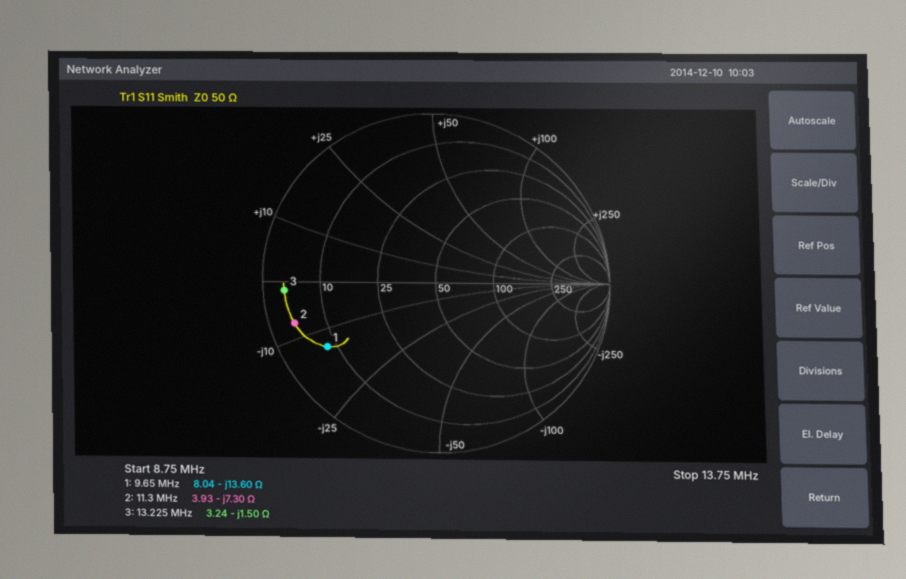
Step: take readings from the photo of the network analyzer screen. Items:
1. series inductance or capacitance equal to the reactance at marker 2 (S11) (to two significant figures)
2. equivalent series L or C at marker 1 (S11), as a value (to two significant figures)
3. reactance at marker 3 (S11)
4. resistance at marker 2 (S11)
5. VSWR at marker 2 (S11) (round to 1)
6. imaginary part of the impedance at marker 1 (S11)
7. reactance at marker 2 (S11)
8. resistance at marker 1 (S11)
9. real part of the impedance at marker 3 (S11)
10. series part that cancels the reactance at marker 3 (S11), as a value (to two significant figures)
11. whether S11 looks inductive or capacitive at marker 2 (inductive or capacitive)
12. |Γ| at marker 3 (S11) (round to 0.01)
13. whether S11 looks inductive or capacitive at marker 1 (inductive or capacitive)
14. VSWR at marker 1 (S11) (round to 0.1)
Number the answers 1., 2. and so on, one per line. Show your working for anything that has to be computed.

1. C = 1/(2π × 11.3 MHz × 7.3 Ω) ≈ 1.9 nF
2. C = 1/(2π × 9.65 MHz × 13.6 Ω) ≈ 1.2 nF
3. -1.50 Ω
4. 3.93 Ω
5. 13
6. -13.60 Ω
7. -7.30 Ω
8. 8.04 Ω
9. 3.24 Ω
10. L = 1.5 Ω/(2π × 13.225 MHz) ≈ 18 nH
11. capacitive
12. 0.88
13. capacitive
14. 6.7
